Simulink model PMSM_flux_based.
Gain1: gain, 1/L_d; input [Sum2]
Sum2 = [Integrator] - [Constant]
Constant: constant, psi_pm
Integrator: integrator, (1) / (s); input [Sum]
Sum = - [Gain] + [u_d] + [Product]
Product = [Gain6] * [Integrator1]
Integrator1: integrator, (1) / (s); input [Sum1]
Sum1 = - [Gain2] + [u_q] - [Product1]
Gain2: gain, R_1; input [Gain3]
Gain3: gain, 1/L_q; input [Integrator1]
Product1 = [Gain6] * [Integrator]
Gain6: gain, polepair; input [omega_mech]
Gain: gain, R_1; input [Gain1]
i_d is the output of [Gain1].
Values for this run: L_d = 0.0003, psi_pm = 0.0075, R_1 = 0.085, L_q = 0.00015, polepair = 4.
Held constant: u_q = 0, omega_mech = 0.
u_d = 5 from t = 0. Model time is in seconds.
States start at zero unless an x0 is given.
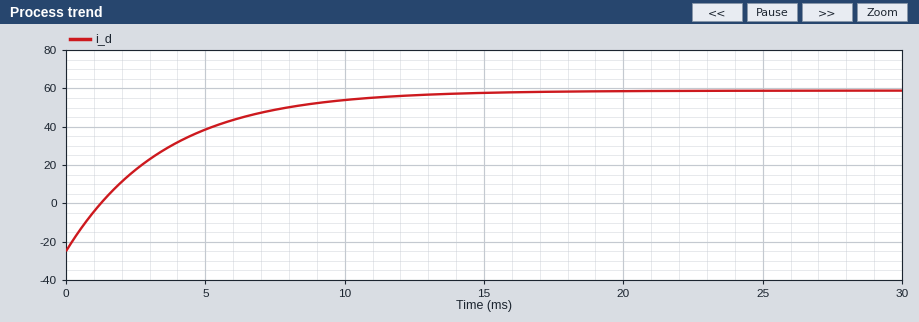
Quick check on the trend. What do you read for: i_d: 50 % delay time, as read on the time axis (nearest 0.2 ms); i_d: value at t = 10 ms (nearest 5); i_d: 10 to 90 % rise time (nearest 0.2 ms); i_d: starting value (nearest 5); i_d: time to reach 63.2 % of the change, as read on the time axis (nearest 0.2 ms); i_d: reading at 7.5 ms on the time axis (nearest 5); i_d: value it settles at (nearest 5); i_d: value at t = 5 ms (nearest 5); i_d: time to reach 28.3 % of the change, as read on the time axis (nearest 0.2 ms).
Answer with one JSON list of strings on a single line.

["2.4 ms", "55", "7.8 ms", "-25", "3.6 ms", "50", "60", "40", "1.2 ms"]
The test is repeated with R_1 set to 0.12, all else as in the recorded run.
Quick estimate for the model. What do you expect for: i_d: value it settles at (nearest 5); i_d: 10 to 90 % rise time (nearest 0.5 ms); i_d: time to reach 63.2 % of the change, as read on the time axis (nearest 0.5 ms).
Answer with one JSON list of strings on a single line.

["40", "5.5 ms", "2.5 ms"]
